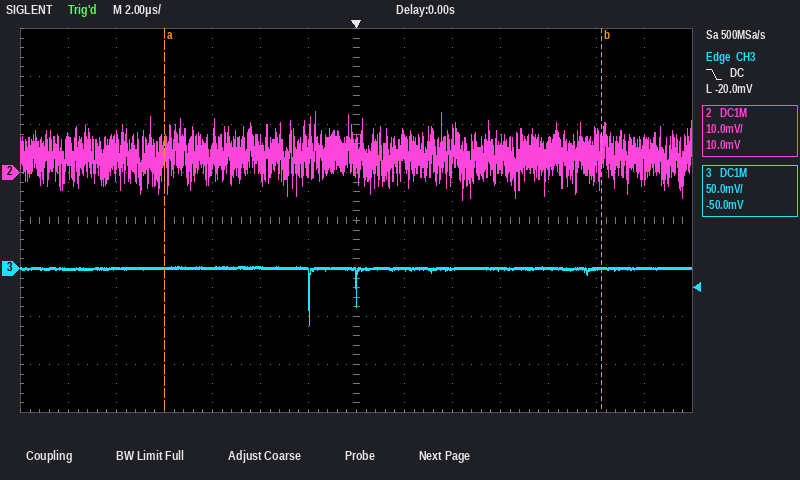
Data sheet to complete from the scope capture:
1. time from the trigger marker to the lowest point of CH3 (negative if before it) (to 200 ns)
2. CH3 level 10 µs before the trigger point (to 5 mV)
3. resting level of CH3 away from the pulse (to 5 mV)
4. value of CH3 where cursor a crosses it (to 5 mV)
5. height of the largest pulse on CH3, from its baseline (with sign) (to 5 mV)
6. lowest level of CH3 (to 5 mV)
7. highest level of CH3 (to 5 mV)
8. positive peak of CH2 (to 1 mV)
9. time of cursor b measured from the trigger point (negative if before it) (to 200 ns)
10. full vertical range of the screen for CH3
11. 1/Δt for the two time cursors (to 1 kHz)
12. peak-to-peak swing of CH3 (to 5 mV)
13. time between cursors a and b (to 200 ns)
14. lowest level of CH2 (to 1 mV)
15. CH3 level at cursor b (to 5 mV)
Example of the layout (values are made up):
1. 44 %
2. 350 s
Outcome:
1. -2.0 µs
2. 0 mV
3. 0 mV
4. 0 mV
5. -60 mV
6. -60 mV
7. 0 mV
8. 13 mV
9. +10.2 µs
10. 400 mV
11. 55 kHz
12. 60 mV
13. 18.2 µs
14. -6 mV
15. 0 mV
